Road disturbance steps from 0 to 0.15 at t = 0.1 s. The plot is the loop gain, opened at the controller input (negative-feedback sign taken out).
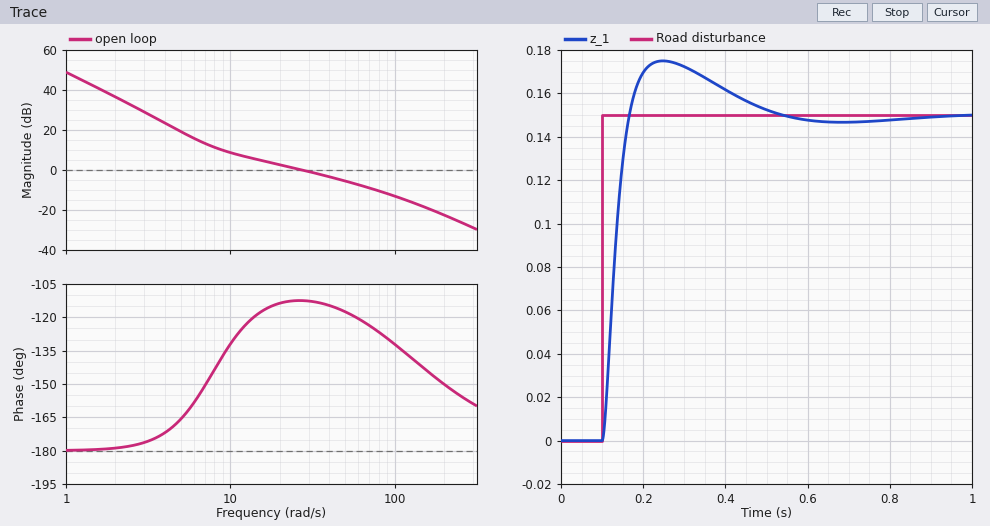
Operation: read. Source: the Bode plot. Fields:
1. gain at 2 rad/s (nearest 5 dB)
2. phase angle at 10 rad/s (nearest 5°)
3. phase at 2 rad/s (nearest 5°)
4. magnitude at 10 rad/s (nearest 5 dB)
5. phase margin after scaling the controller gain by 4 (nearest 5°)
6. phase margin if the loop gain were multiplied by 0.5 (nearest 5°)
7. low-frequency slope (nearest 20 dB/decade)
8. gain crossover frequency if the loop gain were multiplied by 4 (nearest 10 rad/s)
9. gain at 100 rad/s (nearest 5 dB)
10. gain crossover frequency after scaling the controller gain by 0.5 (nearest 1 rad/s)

35 dB
-130°
-180°
10 dB
50°
60°
-40 dB/decade
90 rad/s
-15 dB
13 rad/s
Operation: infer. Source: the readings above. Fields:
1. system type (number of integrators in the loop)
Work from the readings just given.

2
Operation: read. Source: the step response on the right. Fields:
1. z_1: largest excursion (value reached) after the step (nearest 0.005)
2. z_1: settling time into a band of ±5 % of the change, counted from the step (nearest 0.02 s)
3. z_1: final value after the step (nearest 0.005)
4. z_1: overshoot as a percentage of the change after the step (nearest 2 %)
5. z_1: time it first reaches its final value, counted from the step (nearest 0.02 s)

0.175
0.34 s
0.150
16 %
0.06 s
